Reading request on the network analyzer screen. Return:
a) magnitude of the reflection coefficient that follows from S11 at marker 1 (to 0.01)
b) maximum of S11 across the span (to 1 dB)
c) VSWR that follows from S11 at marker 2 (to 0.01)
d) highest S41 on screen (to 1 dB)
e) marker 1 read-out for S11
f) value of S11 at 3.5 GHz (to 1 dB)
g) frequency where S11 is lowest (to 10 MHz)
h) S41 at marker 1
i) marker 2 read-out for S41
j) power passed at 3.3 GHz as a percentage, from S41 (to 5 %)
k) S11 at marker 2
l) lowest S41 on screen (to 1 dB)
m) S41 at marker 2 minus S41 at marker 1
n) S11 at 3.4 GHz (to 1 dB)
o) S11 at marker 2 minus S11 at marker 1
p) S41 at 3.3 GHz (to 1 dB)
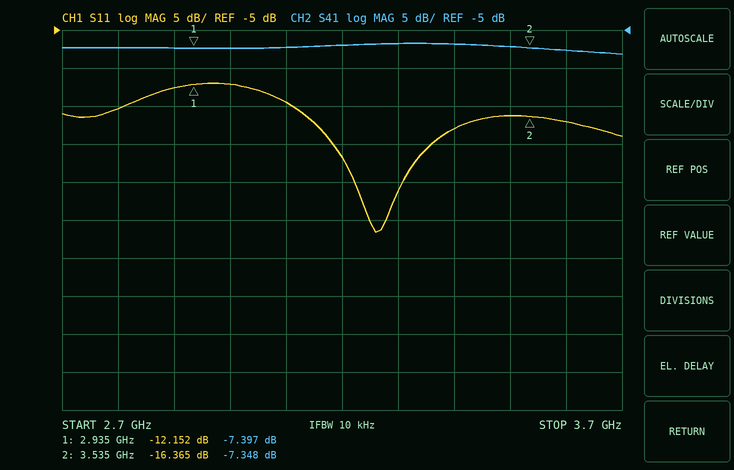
0.25
-12 dB
1.36
-7 dB
-12.152 dB
-16 dB
3.26 GHz
-7.397 dB
-7.348 dB
20 %
-16.365 dB
-8 dB
0.049 dB
-18 dB
-4.213 dB
-7 dB
